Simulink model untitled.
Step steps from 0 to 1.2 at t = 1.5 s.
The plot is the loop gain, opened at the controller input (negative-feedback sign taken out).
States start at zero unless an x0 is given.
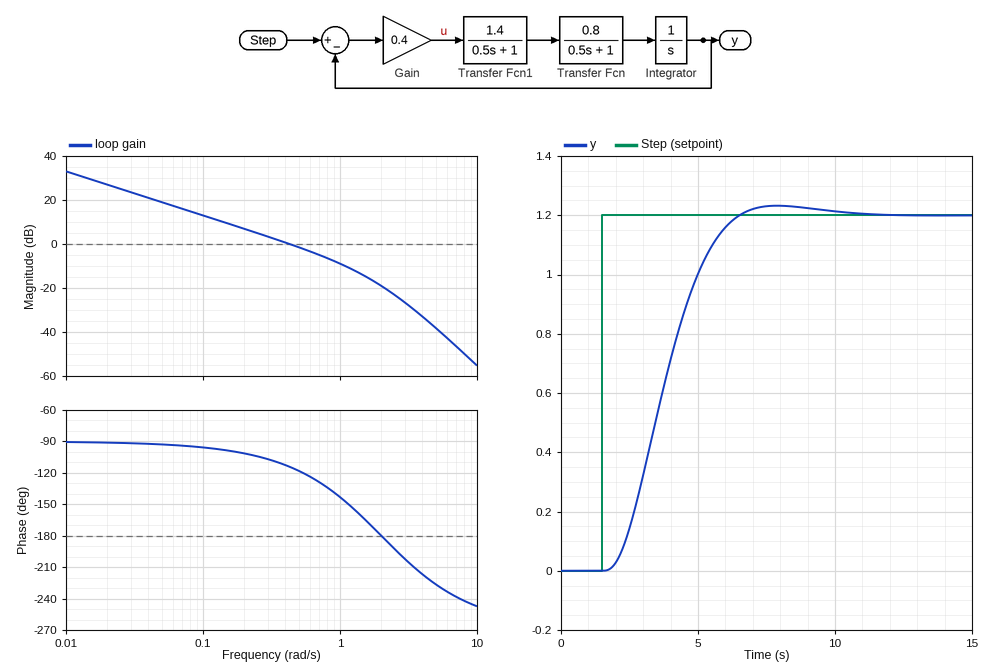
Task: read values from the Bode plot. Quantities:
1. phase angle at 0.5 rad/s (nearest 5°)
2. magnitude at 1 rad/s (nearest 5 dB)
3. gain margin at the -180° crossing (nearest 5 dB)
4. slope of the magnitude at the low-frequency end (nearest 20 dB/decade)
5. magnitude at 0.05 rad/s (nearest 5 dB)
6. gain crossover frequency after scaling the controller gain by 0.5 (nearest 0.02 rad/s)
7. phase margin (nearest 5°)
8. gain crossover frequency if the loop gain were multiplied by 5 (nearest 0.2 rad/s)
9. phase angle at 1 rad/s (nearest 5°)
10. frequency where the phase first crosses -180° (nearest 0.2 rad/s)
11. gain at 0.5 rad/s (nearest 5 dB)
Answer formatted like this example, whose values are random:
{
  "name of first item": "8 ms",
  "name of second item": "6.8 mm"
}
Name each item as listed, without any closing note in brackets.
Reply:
{
  "phase angle at 0.5 rad/s": "-120°",
  "magnitude at 1 rad/s": "-10 dB",
  "gain margin at the -180° crossing": "20 dB",
  "slope of the magnitude at the low-frequency end": "-20 dB/decade",
  "magnitude at 0.05 rad/s": "20 dB",
  "gain crossover frequency after scaling the controller gain by 0.5": "0.22 rad/s",
  "phase margin": "65°",
  "gain crossover frequency if the loop gain were multiplied by 5": "1.4 rad/s",
  "phase angle at 1 rad/s": "-145°",
  "frequency where the phase first crosses -180°": "2.0 rad/s",
  "gain at 0.5 rad/s": "0 dB"
}
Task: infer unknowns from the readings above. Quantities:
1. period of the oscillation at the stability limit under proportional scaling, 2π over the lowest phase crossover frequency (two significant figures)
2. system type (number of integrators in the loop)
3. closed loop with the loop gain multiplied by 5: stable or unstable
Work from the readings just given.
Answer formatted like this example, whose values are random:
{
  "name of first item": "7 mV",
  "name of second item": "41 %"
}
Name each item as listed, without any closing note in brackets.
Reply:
{
  "period of the oscillation at the stability limit under proportional scaling, 2π over the lowest phase crossover frequency": "3.1 s",
  "system type": "1",
  "closed loop with the loop gain multiplied by 5: stable or unstable": "stable"
}
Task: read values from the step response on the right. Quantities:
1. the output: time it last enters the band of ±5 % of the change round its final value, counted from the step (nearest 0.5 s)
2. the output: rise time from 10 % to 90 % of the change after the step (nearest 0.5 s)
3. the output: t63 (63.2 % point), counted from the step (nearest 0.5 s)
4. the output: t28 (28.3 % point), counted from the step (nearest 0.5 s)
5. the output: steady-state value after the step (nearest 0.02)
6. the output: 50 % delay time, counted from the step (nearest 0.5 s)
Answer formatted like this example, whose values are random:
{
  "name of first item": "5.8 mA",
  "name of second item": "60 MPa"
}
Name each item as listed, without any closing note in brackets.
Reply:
{
  "the output: time it last enters the band of ±5 % of the change round its final value, counted from the step": "4.5 s",
  "the output: rise time from 10 % to 90 % of the change after the step": "3.0 s",
  "the output: t63 (63.2 % point), counted from the step": "2.5 s",
  "the output: t28 (28.3 % point), counted from the step": "1.5 s",
  "the output: steady-state value after the step": "1.20",
  "the output: 50 % delay time, counted from the step": "2.0 s"
}
